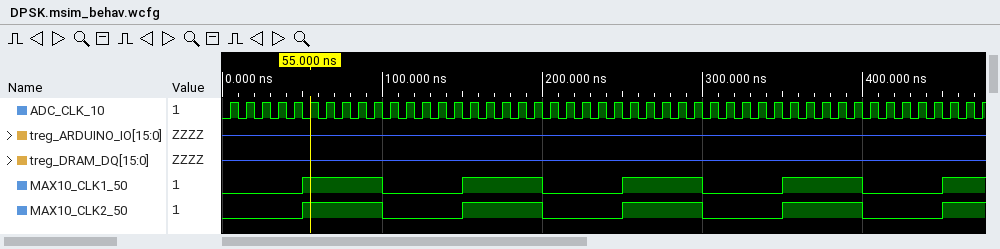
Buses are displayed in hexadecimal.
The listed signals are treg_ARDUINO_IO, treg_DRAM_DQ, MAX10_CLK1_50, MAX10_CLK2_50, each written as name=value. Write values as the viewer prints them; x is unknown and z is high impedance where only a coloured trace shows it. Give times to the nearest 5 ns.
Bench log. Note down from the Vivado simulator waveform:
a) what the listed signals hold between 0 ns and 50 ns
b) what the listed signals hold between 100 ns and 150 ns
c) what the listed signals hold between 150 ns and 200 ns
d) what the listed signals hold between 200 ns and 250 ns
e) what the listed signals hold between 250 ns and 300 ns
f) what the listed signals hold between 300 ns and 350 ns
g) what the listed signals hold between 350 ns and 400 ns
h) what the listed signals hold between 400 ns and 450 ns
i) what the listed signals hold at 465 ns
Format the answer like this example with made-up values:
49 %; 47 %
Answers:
treg_ARDUINO_IO=z, treg_DRAM_DQ=z, MAX10_CLK1_50=0, MAX10_CLK2_50=0; treg_ARDUINO_IO=z, treg_DRAM_DQ=z, MAX10_CLK1_50=0, MAX10_CLK2_50=0; treg_ARDUINO_IO=z, treg_DRAM_DQ=z, MAX10_CLK1_50=1, MAX10_CLK2_50=1; treg_ARDUINO_IO=z, treg_DRAM_DQ=z, MAX10_CLK1_50=0, MAX10_CLK2_50=0; treg_ARDUINO_IO=z, treg_DRAM_DQ=z, MAX10_CLK1_50=1, MAX10_CLK2_50=1; treg_ARDUINO_IO=z, treg_DRAM_DQ=z, MAX10_CLK1_50=0, MAX10_CLK2_50=0; treg_ARDUINO_IO=z, treg_DRAM_DQ=z, MAX10_CLK1_50=1, MAX10_CLK2_50=1; treg_ARDUINO_IO=z, treg_DRAM_DQ=z, MAX10_CLK1_50=0, MAX10_CLK2_50=0; treg_ARDUINO_IO=z, treg_DRAM_DQ=z, MAX10_CLK1_50=1, MAX10_CLK2_50=1
